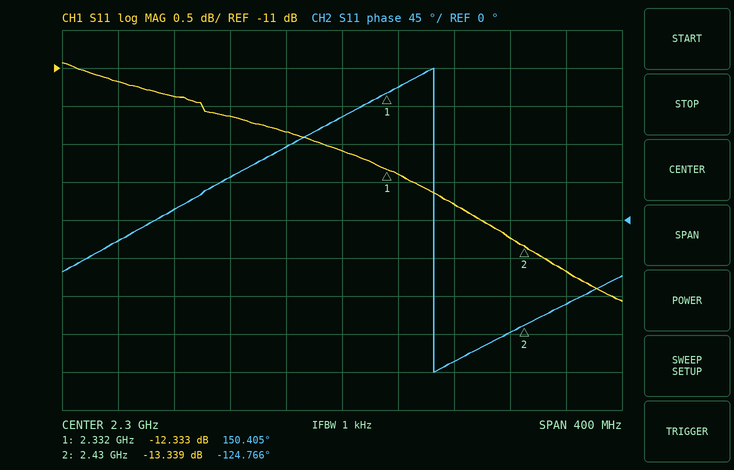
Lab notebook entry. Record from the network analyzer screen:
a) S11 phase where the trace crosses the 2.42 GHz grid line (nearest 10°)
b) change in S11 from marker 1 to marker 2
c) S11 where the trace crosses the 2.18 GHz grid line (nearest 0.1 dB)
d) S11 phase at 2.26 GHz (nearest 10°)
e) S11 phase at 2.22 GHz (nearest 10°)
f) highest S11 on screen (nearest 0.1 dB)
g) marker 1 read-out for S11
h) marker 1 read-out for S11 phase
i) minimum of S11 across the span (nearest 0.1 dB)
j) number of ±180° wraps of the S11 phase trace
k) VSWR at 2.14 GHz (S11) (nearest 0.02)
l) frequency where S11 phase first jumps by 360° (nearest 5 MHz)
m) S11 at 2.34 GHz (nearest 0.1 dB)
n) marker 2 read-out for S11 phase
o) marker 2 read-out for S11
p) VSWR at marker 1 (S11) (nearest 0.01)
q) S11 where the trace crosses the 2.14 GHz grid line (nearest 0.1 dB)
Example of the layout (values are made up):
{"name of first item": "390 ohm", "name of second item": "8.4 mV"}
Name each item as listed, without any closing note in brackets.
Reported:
{"S11 phase where the trace crosses the 2.42 GHz grid line": "-130°", "change in S11 from marker 1 to marker 2": "-1.006 dB", "S11 where the trace crosses the 2.18 GHz grid line": "-11.4 dB", "S11 phase at 2.26 GHz": "90°", "S11 phase at 2.22 GHz": "50°", "highest S11 on screen": "-10.9 dB", "marker 1 read-out for S11": "-12.333 dB", "marker 1 read-out for S11 phase": "150.405°", "minimum of S11 across the span": "-14.1 dB", "number of ±180° wraps of the S11 phase trace": "1", "VSWR at 2.14 GHz (S11)": "1.76", "frequency where S11 phase first jumps by 360°": "2.365 GHz", "S11 at 2.34 GHz": "-12.4 dB", "marker 2 read-out for S11 phase": "-124.766°", "marker 2 read-out for S11": "-13.339 dB", "VSWR at marker 1 (S11)": "1.64", "S11 where the trace crosses the 2.14 GHz grid line": "-11.2 dB"}
